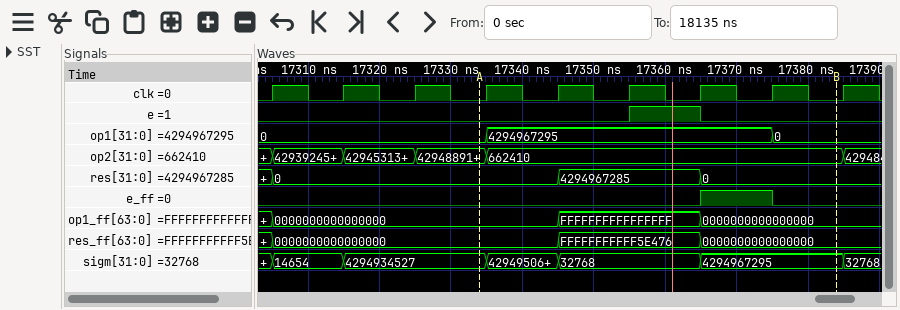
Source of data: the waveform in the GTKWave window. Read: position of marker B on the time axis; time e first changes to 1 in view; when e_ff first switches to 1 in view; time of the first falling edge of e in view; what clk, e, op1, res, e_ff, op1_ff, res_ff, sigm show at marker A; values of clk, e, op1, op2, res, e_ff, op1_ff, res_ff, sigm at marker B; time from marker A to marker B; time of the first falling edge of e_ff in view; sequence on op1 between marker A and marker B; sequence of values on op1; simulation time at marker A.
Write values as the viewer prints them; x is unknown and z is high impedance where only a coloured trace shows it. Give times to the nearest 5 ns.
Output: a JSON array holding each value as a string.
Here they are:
["17385 ns", "17355 ns", "17365 ns", "17365 ns", "clk=0, e=0, op1=0, res=0, e_ff=0, op1_ff=0000000000000000, res_ff=0000000000000000, sigm=4294934527", "clk=0, e=0, op1=0, op2=662410, res=0, e_ff=0, op1_ff=0000000000000000, res_ff=0000000000000000, sigm=4294967295", "50 ns", "17375 ns", "0, 4294967295, 0", "0, 4294967295, 0", "17335 ns"]
